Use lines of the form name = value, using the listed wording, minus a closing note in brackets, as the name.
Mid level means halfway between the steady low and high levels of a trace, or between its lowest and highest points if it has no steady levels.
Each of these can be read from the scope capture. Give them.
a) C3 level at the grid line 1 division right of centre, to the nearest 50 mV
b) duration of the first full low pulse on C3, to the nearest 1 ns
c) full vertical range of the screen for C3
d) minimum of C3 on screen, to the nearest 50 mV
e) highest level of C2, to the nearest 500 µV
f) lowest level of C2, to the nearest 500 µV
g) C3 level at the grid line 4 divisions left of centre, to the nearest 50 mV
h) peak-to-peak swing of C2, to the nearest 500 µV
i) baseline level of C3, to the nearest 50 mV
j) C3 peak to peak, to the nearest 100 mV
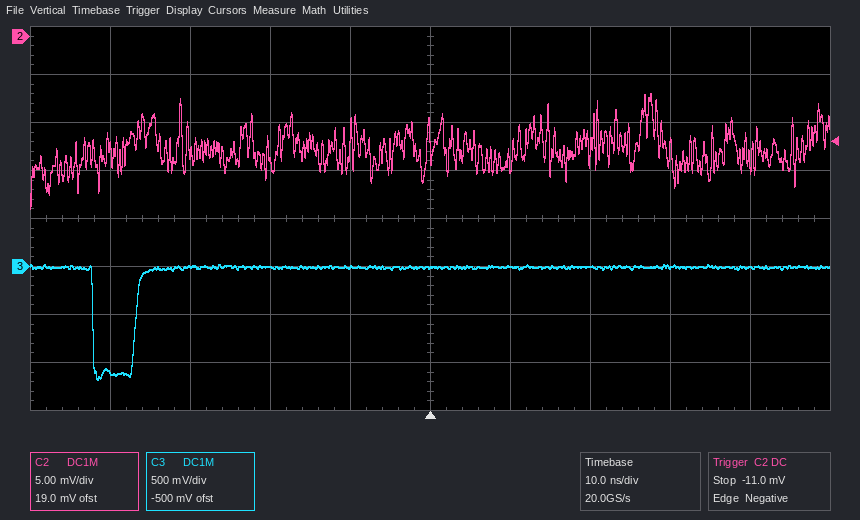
C3 level at the grid line 1 division right of centre, to the nearest 50 mV = 0 mV
duration of the first full low pulse on C3, to the nearest 1 ns = 5 ns
full vertical range of the screen for C3 = 4 V
minimum of C3 on screen, to the nearest 50 mV = -1.20 V
highest level of C2, to the nearest 500 µV = -6.0 mV
lowest level of C2, to the nearest 500 µV = -18.0 mV
C3 level at the grid line 4 divisions left of centre, to the nearest 50 mV = -1.10 V
peak-to-peak swing of C2, to the nearest 500 µV = 12.0 mV
baseline level of C3, to the nearest 50 mV = 0 mV
C3 peak to peak, to the nearest 100 mV = 1.20 V
